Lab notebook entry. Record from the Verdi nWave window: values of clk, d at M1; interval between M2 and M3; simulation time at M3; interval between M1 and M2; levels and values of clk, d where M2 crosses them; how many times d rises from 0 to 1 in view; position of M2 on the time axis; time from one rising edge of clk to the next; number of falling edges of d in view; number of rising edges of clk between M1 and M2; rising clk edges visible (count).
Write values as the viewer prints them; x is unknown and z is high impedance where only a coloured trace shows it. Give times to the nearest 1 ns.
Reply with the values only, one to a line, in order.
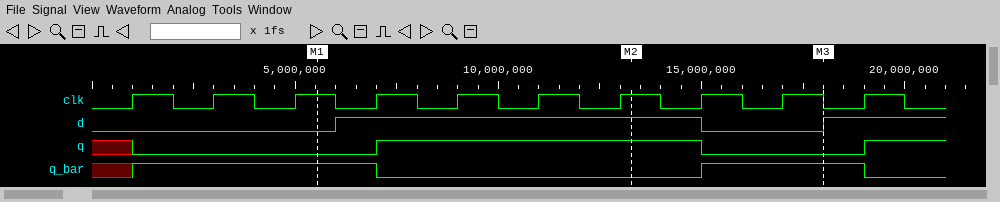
clk=1, d=0
5 ns
18 ns
8 ns
clk=1, d=1
2
13 ns
2 ns
1
4
10
